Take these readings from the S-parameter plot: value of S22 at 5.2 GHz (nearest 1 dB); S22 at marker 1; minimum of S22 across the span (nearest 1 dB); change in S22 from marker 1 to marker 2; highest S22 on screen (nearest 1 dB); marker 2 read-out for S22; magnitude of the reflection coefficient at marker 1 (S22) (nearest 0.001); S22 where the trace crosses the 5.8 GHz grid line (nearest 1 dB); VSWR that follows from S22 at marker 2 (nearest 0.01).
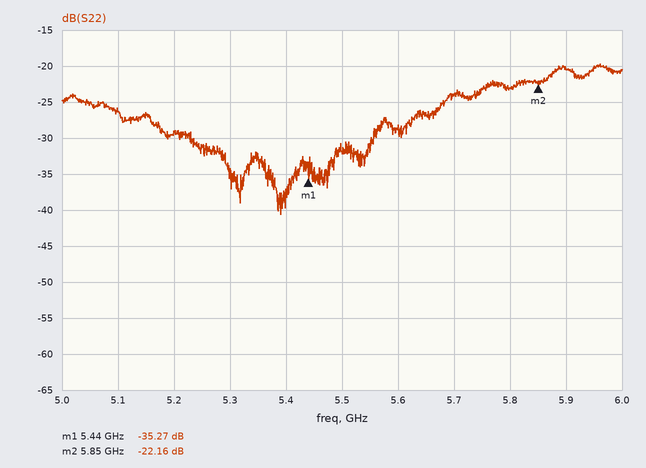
-29 dB
-35.27 dB
-41 dB
13.11 dB
-20 dB
-22.16 dB
0.017
-23 dB
1.17
